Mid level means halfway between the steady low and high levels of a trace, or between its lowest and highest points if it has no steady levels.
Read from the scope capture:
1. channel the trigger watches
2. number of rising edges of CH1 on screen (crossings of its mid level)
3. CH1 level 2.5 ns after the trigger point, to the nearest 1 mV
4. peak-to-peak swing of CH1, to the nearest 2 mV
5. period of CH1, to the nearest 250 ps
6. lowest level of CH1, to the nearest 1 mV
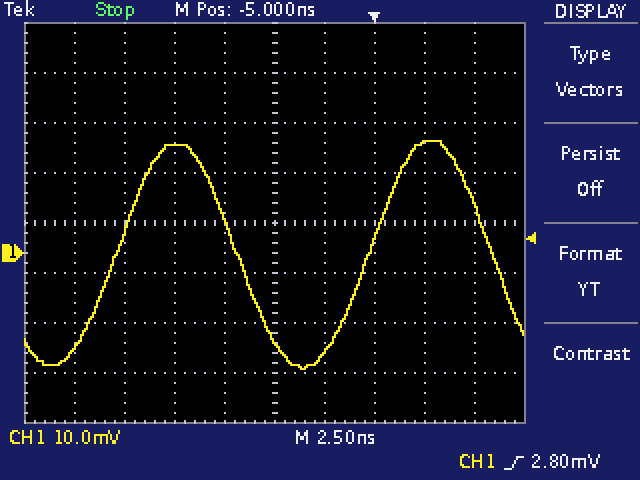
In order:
CH1
2
22 mV
46 mV
12.75 ns
-23 mV
